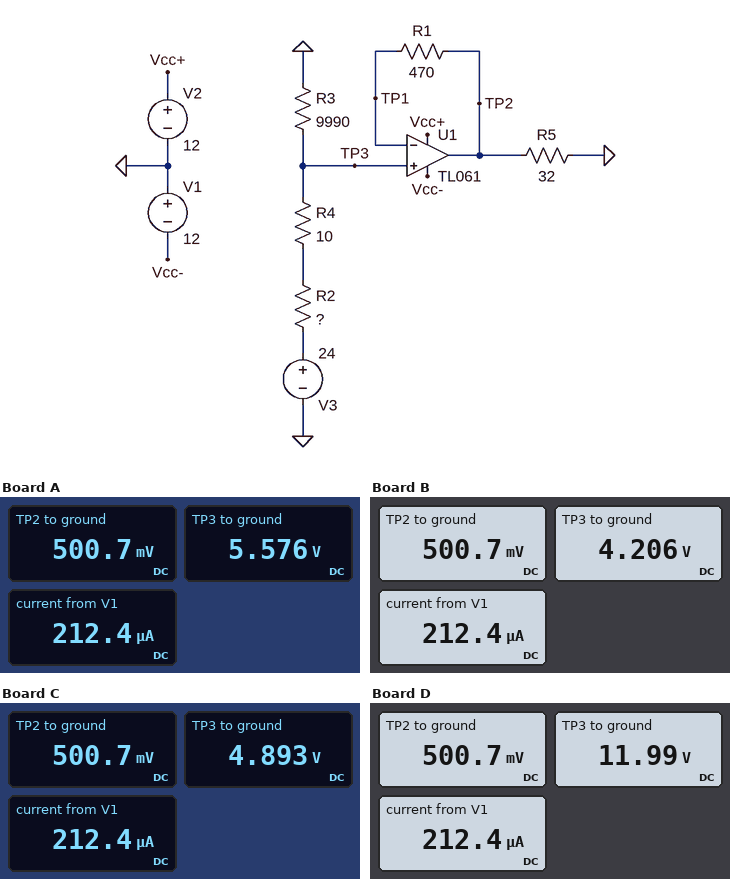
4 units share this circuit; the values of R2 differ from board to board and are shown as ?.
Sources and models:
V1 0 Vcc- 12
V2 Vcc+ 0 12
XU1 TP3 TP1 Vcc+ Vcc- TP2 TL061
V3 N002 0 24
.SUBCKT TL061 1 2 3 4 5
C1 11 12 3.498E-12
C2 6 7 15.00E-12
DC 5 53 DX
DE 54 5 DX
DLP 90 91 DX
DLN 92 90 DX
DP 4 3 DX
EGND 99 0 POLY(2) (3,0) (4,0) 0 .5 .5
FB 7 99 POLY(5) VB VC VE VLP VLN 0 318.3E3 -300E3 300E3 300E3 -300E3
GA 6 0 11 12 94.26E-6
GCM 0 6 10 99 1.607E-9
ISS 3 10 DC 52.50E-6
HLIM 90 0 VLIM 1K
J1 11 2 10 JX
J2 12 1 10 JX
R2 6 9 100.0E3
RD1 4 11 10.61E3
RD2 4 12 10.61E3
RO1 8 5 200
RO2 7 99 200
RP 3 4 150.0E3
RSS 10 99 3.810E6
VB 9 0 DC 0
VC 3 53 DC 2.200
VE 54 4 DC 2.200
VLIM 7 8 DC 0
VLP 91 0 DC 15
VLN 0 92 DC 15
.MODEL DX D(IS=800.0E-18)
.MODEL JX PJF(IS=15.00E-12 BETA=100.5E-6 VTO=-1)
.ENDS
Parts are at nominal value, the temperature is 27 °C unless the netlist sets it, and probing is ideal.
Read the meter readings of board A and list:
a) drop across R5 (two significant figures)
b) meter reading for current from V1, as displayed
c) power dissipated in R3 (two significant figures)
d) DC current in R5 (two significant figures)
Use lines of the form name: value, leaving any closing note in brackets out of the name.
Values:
drop across R5: 500 mV
meter reading for current from V1, as displayed: 212.4 µA
power dissipated in R3: 3.1 mW
DC current in R5: 16 mA
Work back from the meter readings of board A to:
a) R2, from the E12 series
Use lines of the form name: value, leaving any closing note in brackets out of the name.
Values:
R2, from the E12 series: 33 kΩ
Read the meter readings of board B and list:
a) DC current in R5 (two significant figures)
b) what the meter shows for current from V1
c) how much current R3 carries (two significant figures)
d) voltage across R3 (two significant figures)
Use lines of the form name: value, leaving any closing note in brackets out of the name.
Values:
DC current in R5: 16 mA
what the meter shows for current from V1: 212.4 µA
how much current R3 carries: 420 µA
voltage across R3: 4.2 V
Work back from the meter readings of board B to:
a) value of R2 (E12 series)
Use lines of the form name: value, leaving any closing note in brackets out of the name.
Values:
value of R2: 47 kΩ
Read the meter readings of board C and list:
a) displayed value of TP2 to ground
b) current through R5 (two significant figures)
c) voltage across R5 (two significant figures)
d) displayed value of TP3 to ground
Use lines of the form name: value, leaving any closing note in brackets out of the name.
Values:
displayed value of TP2 to ground: 500.7 mV
current through R5: 16 mA
voltage across R5: 500 mV
displayed value of TP3 to ground: 4.893 V
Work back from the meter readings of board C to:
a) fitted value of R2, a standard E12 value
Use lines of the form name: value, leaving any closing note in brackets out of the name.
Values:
fitted value of R2, a standard E12 value: 39 kΩ
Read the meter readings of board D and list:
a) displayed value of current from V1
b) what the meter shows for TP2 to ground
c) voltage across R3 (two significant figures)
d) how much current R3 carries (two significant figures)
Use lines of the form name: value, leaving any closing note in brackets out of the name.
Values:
displayed value of current from V1: 212.4 µA
what the meter shows for TP2 to ground: 500.7 mV
voltage across R3: 12 V
how much current R3 carries: 1.2 mA
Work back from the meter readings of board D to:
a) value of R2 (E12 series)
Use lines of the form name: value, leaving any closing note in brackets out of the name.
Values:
value of R2: 10 kΩ
